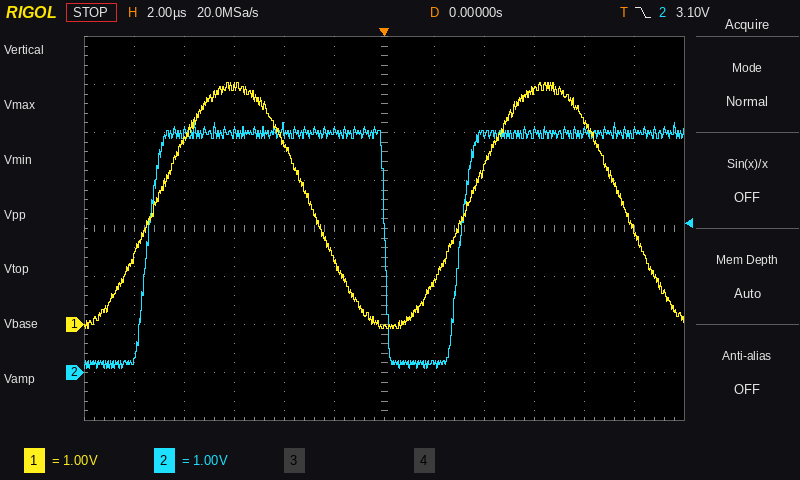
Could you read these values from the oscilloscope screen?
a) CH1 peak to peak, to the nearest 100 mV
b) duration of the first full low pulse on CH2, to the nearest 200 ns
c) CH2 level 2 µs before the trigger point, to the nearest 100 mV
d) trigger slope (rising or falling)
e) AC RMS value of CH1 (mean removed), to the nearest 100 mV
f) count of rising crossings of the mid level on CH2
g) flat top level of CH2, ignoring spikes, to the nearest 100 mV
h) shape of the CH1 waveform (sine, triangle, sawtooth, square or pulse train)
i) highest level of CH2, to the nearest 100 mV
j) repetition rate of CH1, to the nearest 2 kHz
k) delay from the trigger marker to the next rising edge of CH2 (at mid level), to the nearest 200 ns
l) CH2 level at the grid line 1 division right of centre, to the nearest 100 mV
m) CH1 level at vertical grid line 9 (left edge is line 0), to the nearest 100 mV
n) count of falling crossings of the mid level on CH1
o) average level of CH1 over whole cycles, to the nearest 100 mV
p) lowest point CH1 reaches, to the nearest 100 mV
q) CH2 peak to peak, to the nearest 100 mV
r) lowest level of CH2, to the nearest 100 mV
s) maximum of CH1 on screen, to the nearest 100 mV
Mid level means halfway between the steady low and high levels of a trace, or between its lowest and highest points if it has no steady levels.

5.1 V
3.0 µs
5.0 V
falling
1.8 V
2
5.0 V
sine
5.2 V
80 kHz
3.0 µs
200 mV
4.9 V
2
2.5 V
-100 mV
5.1 V
100 mV
5.0 V
